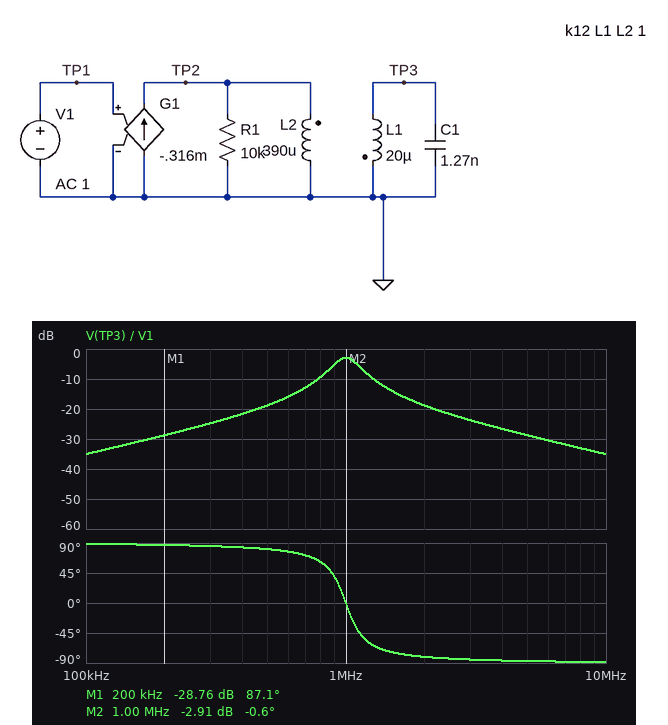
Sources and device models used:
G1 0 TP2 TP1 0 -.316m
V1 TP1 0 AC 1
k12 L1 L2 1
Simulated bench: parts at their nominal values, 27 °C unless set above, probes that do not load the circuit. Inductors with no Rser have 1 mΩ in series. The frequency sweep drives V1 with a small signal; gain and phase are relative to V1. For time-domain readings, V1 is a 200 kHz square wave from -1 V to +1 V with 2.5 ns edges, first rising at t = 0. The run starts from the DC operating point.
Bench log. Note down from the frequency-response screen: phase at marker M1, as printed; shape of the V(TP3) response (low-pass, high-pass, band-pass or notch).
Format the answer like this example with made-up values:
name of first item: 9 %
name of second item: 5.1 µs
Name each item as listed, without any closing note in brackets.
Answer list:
phase at marker M1, as printed: 87.1 deg
shape of the V(TP3) response: band-pass
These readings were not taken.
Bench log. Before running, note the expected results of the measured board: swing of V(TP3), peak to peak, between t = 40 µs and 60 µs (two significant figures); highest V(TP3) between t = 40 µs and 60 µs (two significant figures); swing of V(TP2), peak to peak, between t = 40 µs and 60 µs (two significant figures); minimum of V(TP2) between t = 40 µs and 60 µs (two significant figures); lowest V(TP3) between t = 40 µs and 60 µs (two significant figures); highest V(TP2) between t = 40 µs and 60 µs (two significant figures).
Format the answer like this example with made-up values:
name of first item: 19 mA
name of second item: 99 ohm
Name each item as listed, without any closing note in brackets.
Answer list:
swing of V(TP3), peak to peak, between t = 40 µs and 60 µs: 680 mV
highest V(TP3) between t = 40 µs and 60 µs: 340 mV
swing of V(TP2), peak to peak, between t = 40 µs and 60 µs: 3.0 V
minimum of V(TP2) between t = 40 µs and 60 µs: -1.5 V
lowest V(TP3) between t = 40 µs and 60 µs: -340 mV
highest V(TP2) between t = 40 µs and 60 µs: 1.5 V
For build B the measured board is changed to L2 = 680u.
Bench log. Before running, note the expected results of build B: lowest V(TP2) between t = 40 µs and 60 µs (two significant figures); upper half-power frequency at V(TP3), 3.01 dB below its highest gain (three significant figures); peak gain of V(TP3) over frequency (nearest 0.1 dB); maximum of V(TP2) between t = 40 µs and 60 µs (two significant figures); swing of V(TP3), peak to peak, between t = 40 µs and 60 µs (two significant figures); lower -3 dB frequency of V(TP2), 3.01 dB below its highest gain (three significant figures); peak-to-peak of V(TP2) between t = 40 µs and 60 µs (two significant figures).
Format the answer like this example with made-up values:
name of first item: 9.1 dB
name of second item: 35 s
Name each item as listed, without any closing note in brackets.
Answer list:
lowest V(TP2) between t = 40 µs and 60 µs: -2.1 V
upper half-power frequency at V(TP3), 3.01 dB below its highest gain: 1.23 MHz
peak gain of V(TP3) over frequency: -5.3 dB
maximum of V(TP2) between t = 40 µs and 60 µs: 2.1 V
swing of V(TP3), peak to peak, between t = 40 µs and 60 µs: 710 mV
lower -3 dB frequency of V(TP2), 3.01 dB below its highest gain: 808 kHz
peak-to-peak of V(TP2) between t = 40 µs and 60 µs: 4.1 V
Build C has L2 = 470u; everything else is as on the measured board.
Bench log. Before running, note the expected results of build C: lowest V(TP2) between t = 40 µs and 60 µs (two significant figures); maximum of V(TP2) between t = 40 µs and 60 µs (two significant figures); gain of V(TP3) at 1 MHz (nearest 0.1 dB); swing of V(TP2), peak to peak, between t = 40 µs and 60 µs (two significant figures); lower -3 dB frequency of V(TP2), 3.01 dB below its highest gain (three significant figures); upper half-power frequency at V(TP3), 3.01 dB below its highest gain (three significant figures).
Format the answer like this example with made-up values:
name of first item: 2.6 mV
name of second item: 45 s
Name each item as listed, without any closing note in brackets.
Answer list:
lowest V(TP2) between t = 40 µs and 60 µs: -1.7 V
maximum of V(TP2) between t = 40 µs and 60 µs: 1.7 V
gain of V(TP3) at 1 MHz: -3.7 dB
swing of V(TP2), peak to peak, between t = 40 µs and 60 µs: 3.3 V
lower -3 dB frequency of V(TP2), 3.01 dB below its highest gain: 862 kHz
upper half-power frequency at V(TP3), 3.01 dB below its highest gain: 1.16 MHz
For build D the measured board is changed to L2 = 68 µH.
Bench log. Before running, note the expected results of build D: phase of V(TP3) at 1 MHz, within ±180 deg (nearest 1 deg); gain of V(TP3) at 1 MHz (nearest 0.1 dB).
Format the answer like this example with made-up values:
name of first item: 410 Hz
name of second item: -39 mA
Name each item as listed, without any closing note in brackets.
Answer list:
phase of V(TP3) at 1 MHz, within ±180 deg: -4 deg
gain of V(TP3) at 1 MHz: 4.7 dB
